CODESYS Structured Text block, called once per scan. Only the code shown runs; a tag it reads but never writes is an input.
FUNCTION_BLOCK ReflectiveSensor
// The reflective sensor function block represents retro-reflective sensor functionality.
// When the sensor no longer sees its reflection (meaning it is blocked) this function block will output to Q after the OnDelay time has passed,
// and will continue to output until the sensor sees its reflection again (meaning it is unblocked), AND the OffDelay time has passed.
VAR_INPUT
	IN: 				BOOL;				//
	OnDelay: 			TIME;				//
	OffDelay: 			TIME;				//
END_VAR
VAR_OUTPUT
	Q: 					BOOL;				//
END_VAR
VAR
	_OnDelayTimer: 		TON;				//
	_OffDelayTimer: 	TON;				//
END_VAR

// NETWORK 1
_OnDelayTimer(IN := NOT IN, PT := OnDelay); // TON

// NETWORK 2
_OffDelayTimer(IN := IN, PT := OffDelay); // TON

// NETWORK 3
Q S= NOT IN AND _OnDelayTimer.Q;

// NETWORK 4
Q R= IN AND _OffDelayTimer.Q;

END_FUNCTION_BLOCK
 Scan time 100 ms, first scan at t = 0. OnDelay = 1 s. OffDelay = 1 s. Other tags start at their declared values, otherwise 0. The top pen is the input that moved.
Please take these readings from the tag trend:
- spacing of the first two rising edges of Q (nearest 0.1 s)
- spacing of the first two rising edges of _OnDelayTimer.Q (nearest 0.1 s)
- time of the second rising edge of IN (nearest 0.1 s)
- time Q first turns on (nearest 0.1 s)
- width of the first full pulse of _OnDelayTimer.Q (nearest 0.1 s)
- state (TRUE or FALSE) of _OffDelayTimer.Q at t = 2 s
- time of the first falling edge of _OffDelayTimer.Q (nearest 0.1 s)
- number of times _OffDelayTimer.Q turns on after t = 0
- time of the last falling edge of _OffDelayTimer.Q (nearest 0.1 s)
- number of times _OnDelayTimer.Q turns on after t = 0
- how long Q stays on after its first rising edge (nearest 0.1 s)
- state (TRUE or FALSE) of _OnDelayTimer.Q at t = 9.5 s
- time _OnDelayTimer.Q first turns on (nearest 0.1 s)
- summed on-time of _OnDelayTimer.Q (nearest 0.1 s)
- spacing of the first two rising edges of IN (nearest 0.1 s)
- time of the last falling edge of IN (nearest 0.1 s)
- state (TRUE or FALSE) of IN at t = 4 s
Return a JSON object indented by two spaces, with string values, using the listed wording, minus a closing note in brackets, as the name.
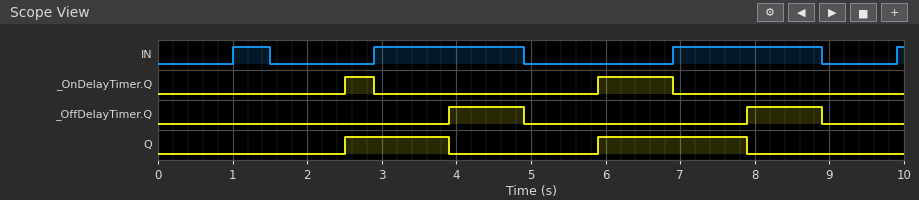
{
  "spacing of the first two rising edges of Q": "3.4 s",
  "spacing of the first two rising edges of _OnDelayTimer.Q": "3.4 s",
  "time of the second rising edge of IN": "2.9 s",
  "time Q first turns on": "2.5 s",
  "width of the first full pulse of _OnDelayTimer.Q": "0.4 s",
  "state (TRUE or FALSE) of _OffDelayTimer.Q at t = 2 s": "FALSE",
  "time of the first falling edge of _OffDelayTimer.Q": "4.9 s",
  "number of times _OffDelayTimer.Q turns on after t = 0": "2",
  "time of the last falling edge of _OffDelayTimer.Q": "8.9 s",
  "number of times _OnDelayTimer.Q turns on after t = 0": "2",
  "how long Q stays on after its first rising edge": "1.4 s",
  "state (TRUE or FALSE) of _OnDelayTimer.Q at t = 9.5 s": "FALSE",
  "time _OnDelayTimer.Q first turns on": "2.5 s",
  "summed on-time of _OnDelayTimer.Q": "1.4 s",
  "spacing of the first two rising edges of IN": "1.9 s",
  "time of the last falling edge of IN": "8.9 s",
  "state (TRUE or FALSE) of IN at t = 4 s": "TRUE"
}
